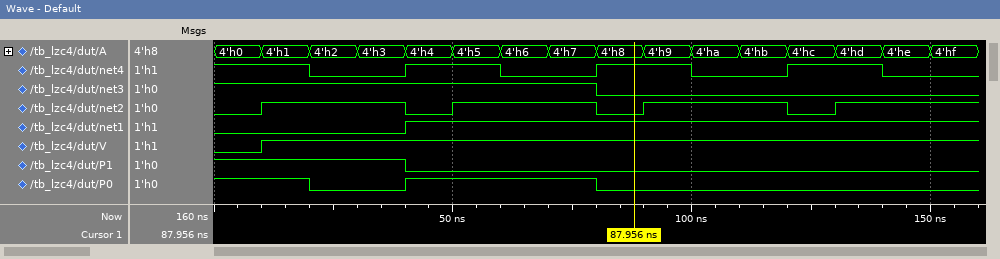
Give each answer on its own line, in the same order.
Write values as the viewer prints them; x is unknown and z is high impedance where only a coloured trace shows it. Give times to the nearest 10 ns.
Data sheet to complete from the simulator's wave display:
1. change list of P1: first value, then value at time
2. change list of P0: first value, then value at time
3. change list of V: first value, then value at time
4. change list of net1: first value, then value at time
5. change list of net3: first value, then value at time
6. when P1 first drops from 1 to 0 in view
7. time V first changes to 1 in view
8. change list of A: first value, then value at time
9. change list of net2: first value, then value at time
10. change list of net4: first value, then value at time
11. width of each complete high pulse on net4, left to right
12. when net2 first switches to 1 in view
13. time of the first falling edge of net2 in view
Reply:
1, 0 at 40 ns
1, 0 at 20 ns, 1 at 40 ns, 0 at 80 ns
0, 1 at 10 ns
0, 1 at 40 ns
1, 0 at 80 ns
40 ns
10 ns
4'h0, 4'h1 at 10 ns, 4'h2 at 20 ns, 4'h3 at 30 ns, 4'h4 at 40 ns, 4'h5 at 50 ns, 4'h6 at 60 ns, 4'h7 at 70 ns, 4'h8 at 80 ns, 4'h9 at 90 ns, 4'ha at 100 ns, 4'hb at 110 ns, 4'hc at 120 ns, 4'hd at 130 ns, 4'he at 140 ns, 4'hf at 150 ns
0, 1 at 10 ns, 0 at 40 ns, 1 at 50 ns, 0 at 80 ns, 1 at 90 ns, 0 at 120 ns, 1 at 130 ns
1, 0 at 20 ns, 1 at 40 ns, 0 at 60 ns, 1 at 80 ns, 0 at 100 ns, 1 at 120 ns, 0 at 140 ns
20 ns, 20 ns, 20 ns
10 ns
40 ns
